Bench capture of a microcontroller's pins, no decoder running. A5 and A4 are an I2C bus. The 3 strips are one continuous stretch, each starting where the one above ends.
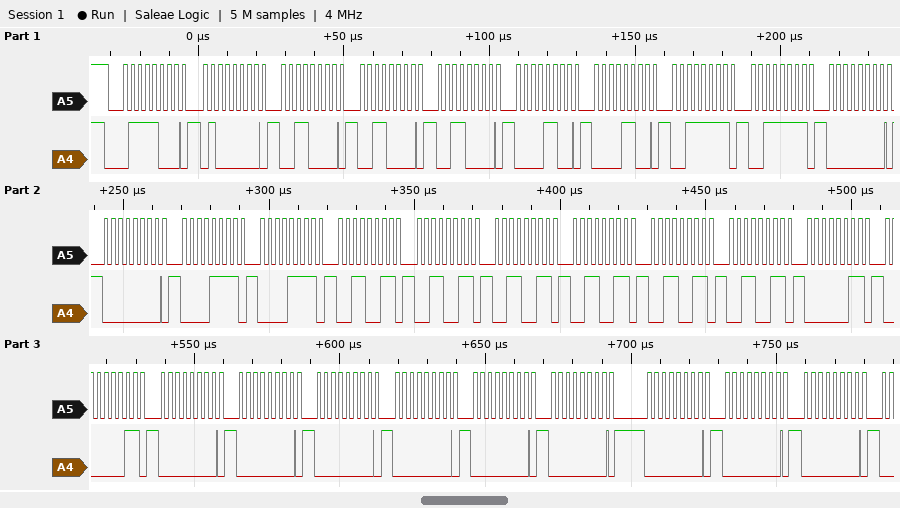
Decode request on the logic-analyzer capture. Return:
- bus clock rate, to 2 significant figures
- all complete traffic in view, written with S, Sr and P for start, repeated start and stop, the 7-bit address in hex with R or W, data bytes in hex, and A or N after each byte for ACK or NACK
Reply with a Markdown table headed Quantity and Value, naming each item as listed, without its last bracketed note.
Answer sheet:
| Quantity | Value |
|---|---|
| bus clock rate, to 2 significant figures | 400 kHz |
| all complete traffic in view, written with S, Sr and P for start, repeated start and stop, the 7-bit address in hex with R or W, data bytes in hex, and A or N after each byte for ACK or NACK | S 3CW A 40 A 30 A 30 A 30 A 0C A 0C A 3F A 3F A 00 A 00 A 0F A 0F A 33 A 33 A 33 A 33 A 33 A 33 A 03 A 03 A 00 A 00 A 00 A 00 A 00 A 00 A 00 A 00 A 00 A |
